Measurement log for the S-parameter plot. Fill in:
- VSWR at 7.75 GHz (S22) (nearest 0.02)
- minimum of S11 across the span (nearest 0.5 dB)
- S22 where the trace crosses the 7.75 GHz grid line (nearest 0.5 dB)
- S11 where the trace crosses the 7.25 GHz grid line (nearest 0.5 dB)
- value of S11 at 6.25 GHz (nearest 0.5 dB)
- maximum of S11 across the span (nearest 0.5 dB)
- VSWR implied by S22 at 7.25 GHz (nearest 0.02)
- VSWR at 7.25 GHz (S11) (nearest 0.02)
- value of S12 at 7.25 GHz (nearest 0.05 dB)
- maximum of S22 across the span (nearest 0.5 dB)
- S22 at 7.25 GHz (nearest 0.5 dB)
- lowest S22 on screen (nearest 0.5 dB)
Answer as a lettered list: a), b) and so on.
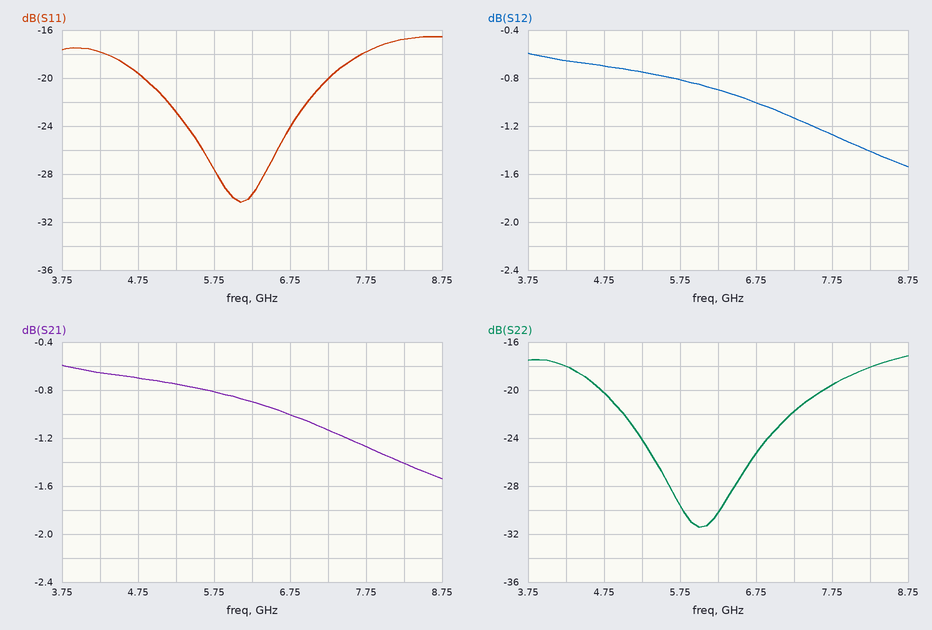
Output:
a) 1.24
b) -30.5 dB
c) -19.5 dB
d) -20.0 dB
e) -29.5 dB
f) -16.5 dB
g) 1.18
h) 1.22
i) -1.15 dB
j) -17.0 dB
k) -22.0 dB
l) -31.5 dB
